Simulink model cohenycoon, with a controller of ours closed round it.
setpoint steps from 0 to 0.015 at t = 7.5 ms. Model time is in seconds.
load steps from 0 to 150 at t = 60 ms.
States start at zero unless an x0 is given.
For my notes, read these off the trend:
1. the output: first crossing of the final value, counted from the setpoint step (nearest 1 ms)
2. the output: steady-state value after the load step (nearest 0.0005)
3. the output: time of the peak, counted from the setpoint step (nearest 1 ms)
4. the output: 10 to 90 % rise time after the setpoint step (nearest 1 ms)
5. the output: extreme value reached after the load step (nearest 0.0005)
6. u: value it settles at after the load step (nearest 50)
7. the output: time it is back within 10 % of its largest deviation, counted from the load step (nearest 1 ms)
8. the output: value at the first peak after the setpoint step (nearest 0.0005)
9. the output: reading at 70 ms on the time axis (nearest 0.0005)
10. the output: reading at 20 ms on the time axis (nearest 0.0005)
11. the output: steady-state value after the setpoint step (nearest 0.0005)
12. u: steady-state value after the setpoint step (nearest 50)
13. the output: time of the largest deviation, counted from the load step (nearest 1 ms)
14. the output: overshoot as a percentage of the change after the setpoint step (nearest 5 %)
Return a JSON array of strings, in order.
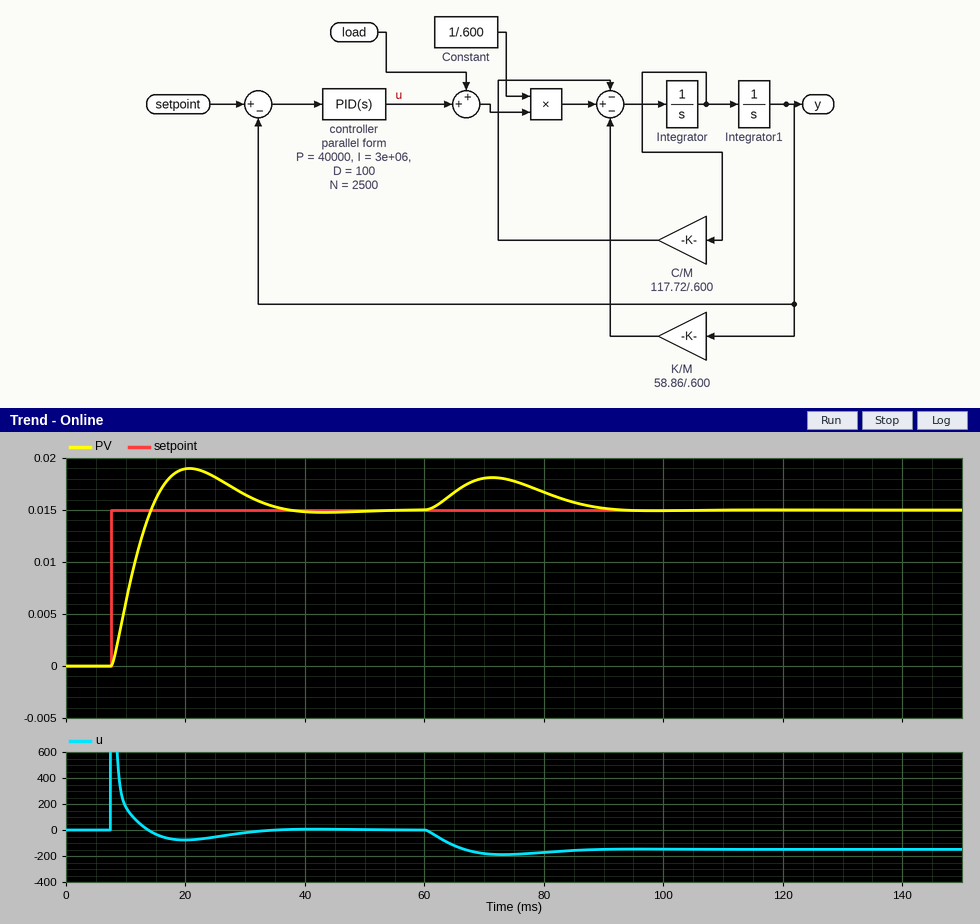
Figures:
["7 ms", "0.0150", "13 ms", "5 ms", "0.0180", "-150", "28 ms", "0.0190", "0.0180", "0.0190", "0.0150", "0", "11 ms", "25 %"]
